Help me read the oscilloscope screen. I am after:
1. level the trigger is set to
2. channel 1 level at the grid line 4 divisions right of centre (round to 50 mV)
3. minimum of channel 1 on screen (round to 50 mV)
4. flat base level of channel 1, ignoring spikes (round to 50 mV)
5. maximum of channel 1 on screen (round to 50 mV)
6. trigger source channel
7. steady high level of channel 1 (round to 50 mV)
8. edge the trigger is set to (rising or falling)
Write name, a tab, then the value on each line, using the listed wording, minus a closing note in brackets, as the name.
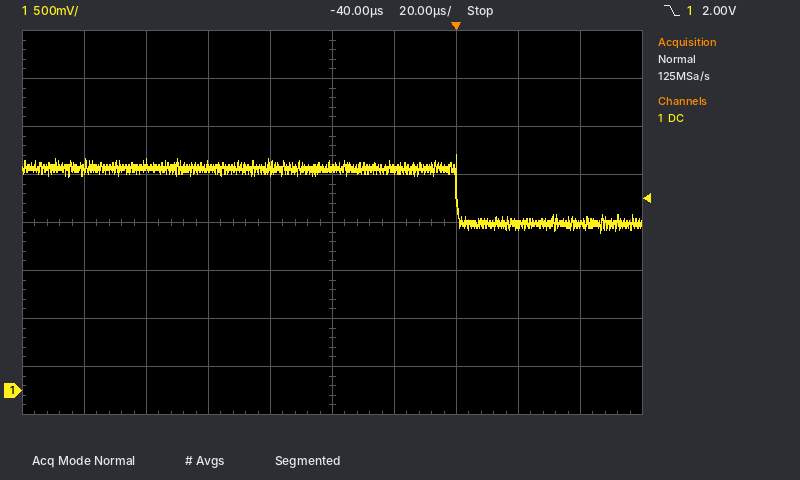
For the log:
level the trigger is set to	2.00 V
channel 1 level at the grid line 4 divisions right of centre	1.75 V
minimum of channel 1 on screen	1.65 V
flat base level of channel 1, ignoring spikes	1.75 V
maximum of channel 1 on screen	2.45 V
trigger source channel	channel 1
steady high level of channel 1	2.30 V
edge the trigger is set to	falling
